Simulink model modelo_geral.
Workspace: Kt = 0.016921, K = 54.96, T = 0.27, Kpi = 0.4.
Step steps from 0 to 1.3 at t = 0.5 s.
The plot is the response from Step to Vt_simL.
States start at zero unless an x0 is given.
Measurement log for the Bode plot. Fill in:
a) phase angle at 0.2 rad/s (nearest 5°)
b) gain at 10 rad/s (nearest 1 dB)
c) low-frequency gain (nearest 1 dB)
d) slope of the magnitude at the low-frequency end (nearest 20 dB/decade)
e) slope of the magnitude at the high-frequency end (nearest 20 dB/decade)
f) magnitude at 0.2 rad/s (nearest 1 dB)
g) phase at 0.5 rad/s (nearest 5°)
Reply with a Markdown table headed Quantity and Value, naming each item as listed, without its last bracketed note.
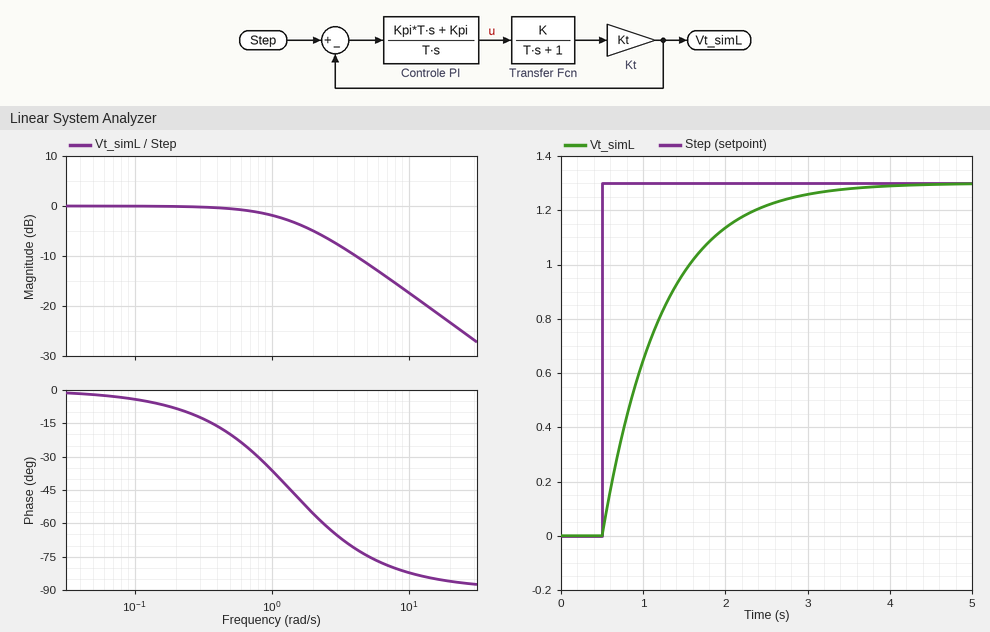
| Quantity | Value |
|---|---|
| phase angle at 0.2 rad/s | -10° |
| gain at 10 rad/s | -17 dB |
| low-frequency gain | 0 dB |
| slope of the magnitude at the low-frequency end | 0 dB/decade |
| slope of the magnitude at the high-frequency end | -20 dB/decade |
| magnitude at 0.2 rad/s | 0 dB |
| phase at 0.5 rad/s | -20° |
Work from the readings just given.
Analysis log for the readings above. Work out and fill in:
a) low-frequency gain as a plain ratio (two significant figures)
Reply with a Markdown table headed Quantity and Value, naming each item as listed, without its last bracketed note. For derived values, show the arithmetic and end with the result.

| Quantity | Value |
|---|---|
| low-frequency gain as a plain ratio | 10^(0 / 20) = 1.0 |
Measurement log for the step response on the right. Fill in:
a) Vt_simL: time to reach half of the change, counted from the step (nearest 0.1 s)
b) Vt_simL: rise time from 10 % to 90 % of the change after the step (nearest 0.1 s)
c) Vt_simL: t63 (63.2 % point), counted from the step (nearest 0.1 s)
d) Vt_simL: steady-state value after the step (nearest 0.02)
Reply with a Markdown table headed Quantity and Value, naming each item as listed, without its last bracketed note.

| Quantity | Value |
|---|---|
| Vt_simL: time to reach half of the change, counted from the step | 0.5 s |
| Vt_simL: rise time from 10 % to 90 % of the change after the step | 1.6 s |
| Vt_simL: t63 (63.2 % point), counted from the step | 0.7 s |
| Vt_simL: steady-state value after the step | 1.30 |
